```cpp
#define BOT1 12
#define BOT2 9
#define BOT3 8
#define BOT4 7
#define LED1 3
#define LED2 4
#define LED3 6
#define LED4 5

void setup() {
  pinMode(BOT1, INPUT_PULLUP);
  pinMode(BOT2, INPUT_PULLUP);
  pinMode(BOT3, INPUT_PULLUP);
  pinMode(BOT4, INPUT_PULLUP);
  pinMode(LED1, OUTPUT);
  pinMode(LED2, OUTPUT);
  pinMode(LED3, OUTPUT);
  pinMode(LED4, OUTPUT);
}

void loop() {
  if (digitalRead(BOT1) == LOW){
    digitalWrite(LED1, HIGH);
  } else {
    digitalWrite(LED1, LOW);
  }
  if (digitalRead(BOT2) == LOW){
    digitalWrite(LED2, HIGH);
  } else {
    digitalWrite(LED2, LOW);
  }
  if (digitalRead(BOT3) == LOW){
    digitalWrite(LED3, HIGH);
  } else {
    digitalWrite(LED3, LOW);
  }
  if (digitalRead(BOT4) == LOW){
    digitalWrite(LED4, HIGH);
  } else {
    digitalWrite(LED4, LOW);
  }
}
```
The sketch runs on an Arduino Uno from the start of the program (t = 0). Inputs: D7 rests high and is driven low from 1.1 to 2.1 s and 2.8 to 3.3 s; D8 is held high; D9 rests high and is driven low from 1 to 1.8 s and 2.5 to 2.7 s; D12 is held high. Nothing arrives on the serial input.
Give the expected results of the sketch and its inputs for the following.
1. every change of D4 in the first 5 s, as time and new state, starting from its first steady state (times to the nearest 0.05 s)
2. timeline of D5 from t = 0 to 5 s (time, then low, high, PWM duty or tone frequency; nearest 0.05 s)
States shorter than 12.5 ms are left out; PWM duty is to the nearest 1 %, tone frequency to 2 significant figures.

0 s low; 1 s high; 1.8 s low; 2.5 s high; 2.7 s low
0 s low; 1.1 s high; 2.1 s low; 2.8 s high; 3.3 s low
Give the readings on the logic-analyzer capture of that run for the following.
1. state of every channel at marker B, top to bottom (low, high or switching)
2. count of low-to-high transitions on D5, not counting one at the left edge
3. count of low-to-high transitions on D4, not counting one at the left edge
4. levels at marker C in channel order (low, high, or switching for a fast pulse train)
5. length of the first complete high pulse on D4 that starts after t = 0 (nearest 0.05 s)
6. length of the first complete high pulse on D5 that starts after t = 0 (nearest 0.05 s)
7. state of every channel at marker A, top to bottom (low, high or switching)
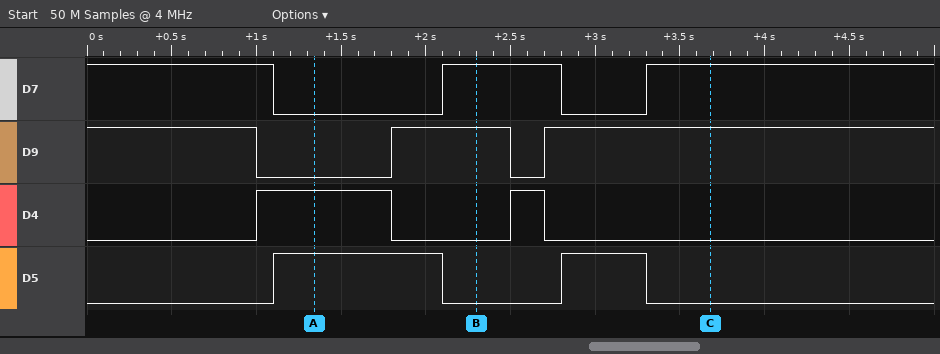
D7 high, D9 high, D4 low, D5 low
2
2
D7 high, D9 high, D4 low, D5 low
0.80 s
1.00 s
D7 low, D9 low, D4 high, D5 high
